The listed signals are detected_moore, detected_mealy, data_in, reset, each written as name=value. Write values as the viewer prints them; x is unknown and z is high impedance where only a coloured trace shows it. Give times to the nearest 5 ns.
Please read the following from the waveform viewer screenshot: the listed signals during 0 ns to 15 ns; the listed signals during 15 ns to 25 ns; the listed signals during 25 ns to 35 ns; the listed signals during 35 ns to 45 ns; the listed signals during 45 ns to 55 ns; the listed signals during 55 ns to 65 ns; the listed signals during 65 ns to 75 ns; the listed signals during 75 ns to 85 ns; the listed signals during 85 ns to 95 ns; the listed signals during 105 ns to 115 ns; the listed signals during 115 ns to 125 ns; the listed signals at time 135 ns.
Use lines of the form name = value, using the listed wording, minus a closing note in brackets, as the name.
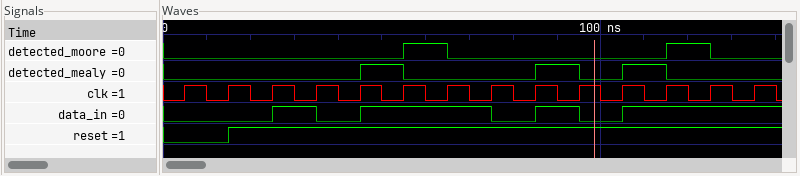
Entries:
the listed signals during 0 ns to 15 ns = detected_moore=0, detected_mealy=0, data_in=0, reset=0
the listed signals during 15 ns to 25 ns = detected_moore=0, detected_mealy=0, data_in=0, reset=1
the listed signals during 25 ns to 35 ns = detected_moore=0, detected_mealy=0, data_in=1, reset=1
the listed signals during 35 ns to 45 ns = detected_moore=0, detected_mealy=0, data_in=0, reset=1
the listed signals during 45 ns to 55 ns = detected_moore=0, detected_mealy=1, data_in=1, reset=1
the listed signals during 55 ns to 65 ns = detected_moore=1, detected_mealy=0, data_in=1, reset=1
the listed signals during 65 ns to 75 ns = detected_moore=0, detected_mealy=0, data_in=1, reset=1
the listed signals during 75 ns to 85 ns = detected_moore=0, detected_mealy=0, data_in=0, reset=1
the listed signals during 85 ns to 95 ns = detected_moore=0, detected_mealy=1, data_in=1, reset=1
the listed signals during 105 ns to 115 ns = detected_moore=0, detected_mealy=1, data_in=1, reset=1
the listed signals during 115 ns to 125 ns = detected_moore=1, detected_mealy=0, data_in=1, reset=1
the listed signals at time 135 ns = detected_moore=0, detected_mealy=0, data_in=1, reset=1
